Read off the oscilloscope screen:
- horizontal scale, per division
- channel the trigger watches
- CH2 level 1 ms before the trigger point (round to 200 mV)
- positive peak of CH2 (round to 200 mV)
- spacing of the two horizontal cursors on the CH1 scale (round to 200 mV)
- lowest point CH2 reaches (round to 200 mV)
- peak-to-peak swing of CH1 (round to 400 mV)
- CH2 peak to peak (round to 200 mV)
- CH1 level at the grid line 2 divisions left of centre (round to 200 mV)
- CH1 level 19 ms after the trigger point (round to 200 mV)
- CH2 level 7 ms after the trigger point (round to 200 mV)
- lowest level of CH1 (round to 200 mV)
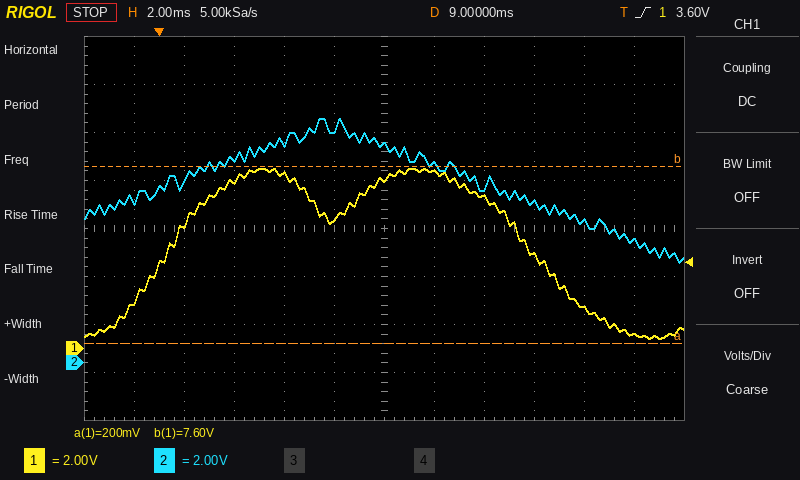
2 ms
CH1
6.8 V
10.2 V
7.4 V
4.2 V
7.2 V
6.0 V
7.2 V
600 mV
9.8 V
400 mV
